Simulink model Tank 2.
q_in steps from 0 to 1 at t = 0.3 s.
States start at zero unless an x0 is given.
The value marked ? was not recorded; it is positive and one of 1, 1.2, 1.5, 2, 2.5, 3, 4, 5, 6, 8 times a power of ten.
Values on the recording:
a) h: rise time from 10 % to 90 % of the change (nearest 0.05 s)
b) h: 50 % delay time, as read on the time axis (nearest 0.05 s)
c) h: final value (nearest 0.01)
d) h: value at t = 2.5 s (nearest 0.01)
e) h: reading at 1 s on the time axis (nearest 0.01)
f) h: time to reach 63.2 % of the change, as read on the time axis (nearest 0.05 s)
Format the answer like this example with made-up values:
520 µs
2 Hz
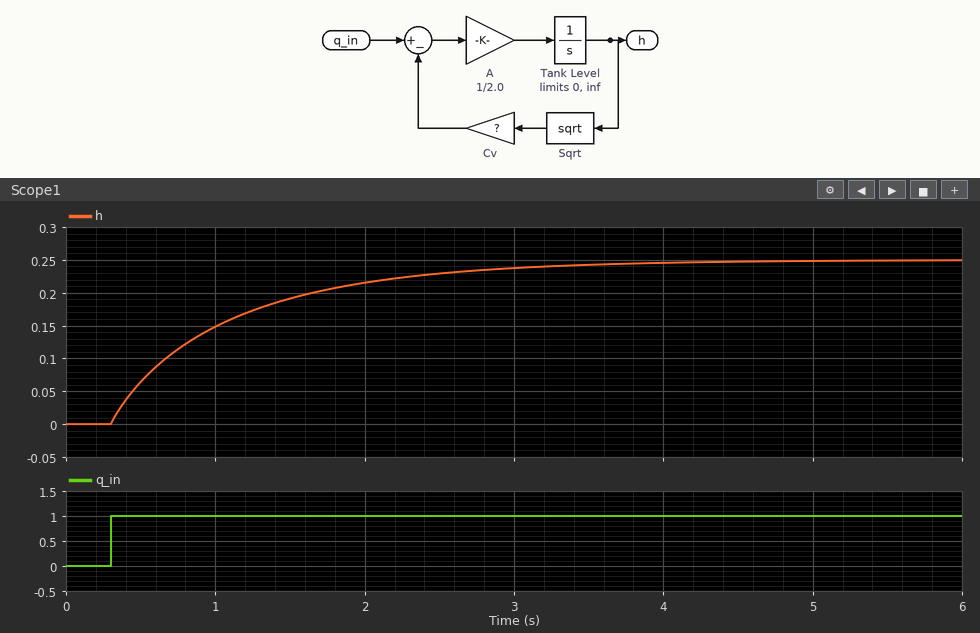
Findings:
1.95 s
0.80 s
0.25
0.23
0.15
1.10 s
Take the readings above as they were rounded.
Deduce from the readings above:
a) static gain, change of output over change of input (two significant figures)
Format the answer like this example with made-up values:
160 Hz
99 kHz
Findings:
0.25
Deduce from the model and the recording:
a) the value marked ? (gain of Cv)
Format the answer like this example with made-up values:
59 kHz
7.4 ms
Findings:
2
